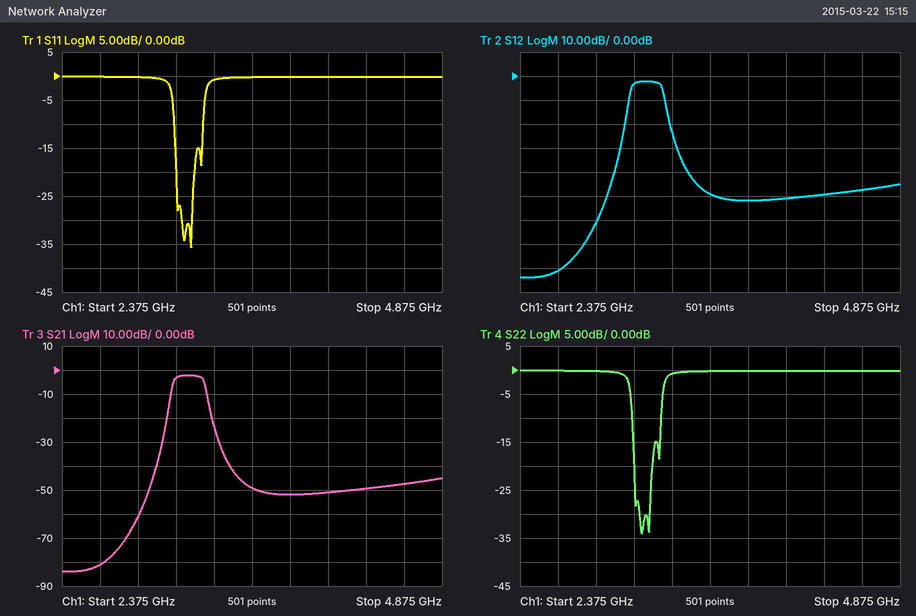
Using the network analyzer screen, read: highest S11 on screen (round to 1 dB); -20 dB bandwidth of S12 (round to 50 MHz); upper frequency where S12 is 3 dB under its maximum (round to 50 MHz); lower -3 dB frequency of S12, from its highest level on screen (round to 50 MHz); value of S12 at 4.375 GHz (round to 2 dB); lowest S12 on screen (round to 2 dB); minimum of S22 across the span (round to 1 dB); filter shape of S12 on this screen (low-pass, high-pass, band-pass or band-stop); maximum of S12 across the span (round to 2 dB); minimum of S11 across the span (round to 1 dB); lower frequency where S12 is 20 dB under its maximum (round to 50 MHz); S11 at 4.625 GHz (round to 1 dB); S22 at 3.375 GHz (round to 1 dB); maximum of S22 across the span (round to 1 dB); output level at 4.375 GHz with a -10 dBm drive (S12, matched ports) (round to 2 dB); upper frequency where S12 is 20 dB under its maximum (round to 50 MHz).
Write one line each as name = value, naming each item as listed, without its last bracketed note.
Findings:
highest S11 on screen = 0 dB
-20 dB bandwidth of S12 = 300 MHz
upper frequency where S12 is 3 dB under its maximum = 3.30 GHz
lower -3 dB frequency of S12, from its highest level on screen = 3.10 GHz
value of S12 at 4.375 GHz = -50 dB
lowest S12 on screen = -84 dB
minimum of S22 across the span = -34 dB
filter shape of S12 on this screen = band-pass
maximum of S12 across the span = -2 dB
minimum of S11 across the span = -36 dB
lower frequency where S12 is 20 dB under its maximum = 3.05 GHz
S11 at 4.625 GHz = 0 dB
S22 at 3.375 GHz = -1 dB
maximum of S22 across the span = 0 dB
output level at 4.375 GHz with a -10 dBm drive (S12, matched ports) = -60 dBm
upper frequency where S12 is 20 dB under its maximum = 3.35 GHz
